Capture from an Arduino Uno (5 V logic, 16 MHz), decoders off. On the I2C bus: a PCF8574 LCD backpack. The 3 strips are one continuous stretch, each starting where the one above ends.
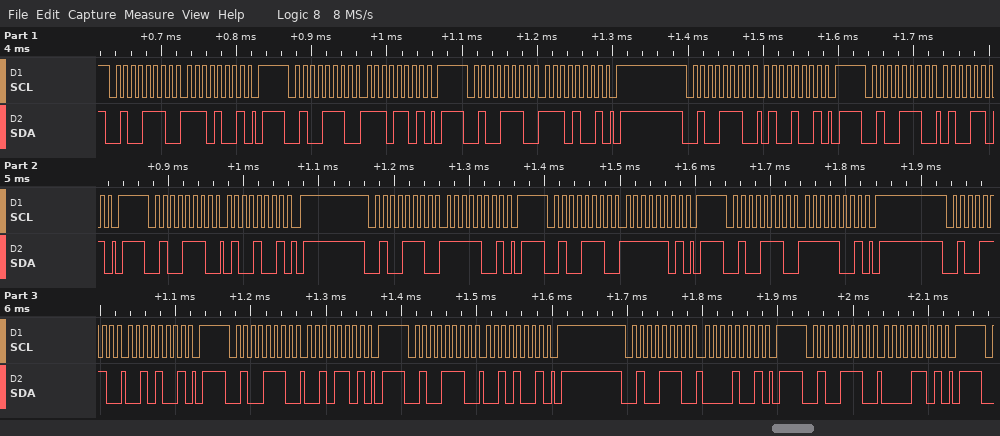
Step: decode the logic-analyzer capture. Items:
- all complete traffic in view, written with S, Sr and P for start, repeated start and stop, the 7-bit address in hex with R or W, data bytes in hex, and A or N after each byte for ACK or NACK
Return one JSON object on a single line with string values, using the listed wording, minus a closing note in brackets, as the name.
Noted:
{"all complete traffic in view, written with S, Sr and P for start, repeated start and stop, the 7-bit address in hex with R or W, data bytes in hex, and A or N after each byte for ACK or NACK": "S 27W A E9 A P S 27W A ED A P S 27W A E9 A P S 27W A 49 A P S 27W A 4D A P S 27W A 49 A P S 27W A F9 A P S 27W A FD A P S 27W A F9 A P S 27W A 29 A P S 27W A 2D A P S 27W A 29 A P S 27W A 09 A P S 27W A 0D A P"}
